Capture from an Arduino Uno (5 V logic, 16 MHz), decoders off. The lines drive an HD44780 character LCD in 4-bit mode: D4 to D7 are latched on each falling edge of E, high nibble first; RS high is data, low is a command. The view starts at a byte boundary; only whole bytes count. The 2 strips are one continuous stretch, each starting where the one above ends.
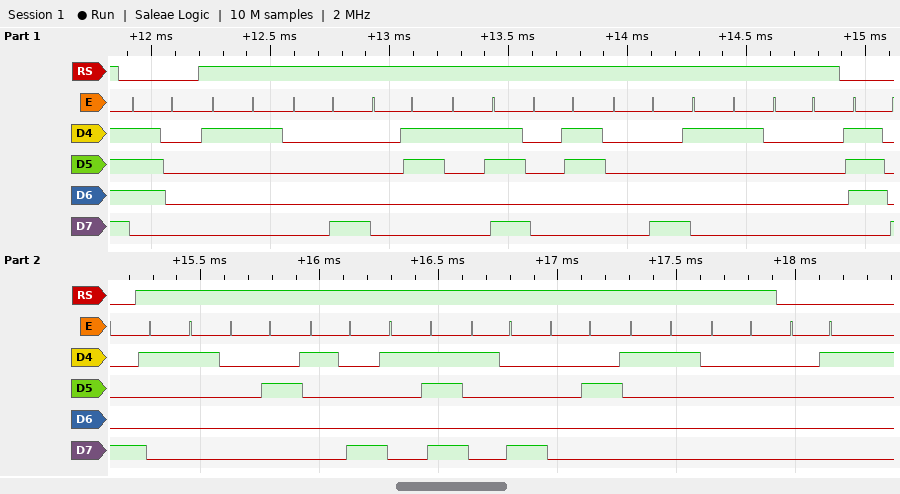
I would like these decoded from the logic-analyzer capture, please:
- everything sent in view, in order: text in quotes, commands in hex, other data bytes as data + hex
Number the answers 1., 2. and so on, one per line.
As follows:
1. 0x70 data 11 08 03 1B 03 08 11 00 0x78 data 11 02 18 1B 18 02 11 00 0x01
